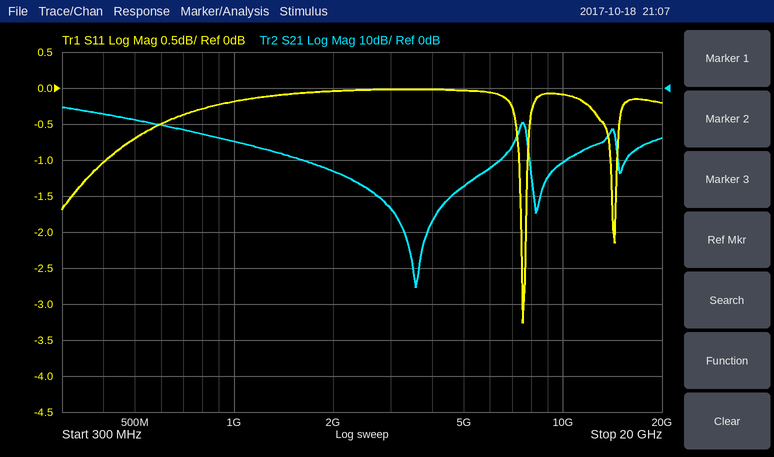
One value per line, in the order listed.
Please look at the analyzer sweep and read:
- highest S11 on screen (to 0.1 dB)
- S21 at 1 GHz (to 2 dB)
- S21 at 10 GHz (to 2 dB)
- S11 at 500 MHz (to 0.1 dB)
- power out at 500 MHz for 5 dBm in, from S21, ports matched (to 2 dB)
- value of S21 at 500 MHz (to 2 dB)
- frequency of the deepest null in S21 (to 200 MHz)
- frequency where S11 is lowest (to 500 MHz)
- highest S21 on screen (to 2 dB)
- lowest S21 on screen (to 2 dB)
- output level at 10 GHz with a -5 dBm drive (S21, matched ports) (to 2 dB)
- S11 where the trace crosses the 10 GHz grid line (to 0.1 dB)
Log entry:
0.0 dB
-14 dB
-20 dB
-0.7 dB
-4 dBm
-8 dB
3.6 GHz
7.5 GHz
-6 dB
-56 dB
-26 dBm
-0.1 dB
